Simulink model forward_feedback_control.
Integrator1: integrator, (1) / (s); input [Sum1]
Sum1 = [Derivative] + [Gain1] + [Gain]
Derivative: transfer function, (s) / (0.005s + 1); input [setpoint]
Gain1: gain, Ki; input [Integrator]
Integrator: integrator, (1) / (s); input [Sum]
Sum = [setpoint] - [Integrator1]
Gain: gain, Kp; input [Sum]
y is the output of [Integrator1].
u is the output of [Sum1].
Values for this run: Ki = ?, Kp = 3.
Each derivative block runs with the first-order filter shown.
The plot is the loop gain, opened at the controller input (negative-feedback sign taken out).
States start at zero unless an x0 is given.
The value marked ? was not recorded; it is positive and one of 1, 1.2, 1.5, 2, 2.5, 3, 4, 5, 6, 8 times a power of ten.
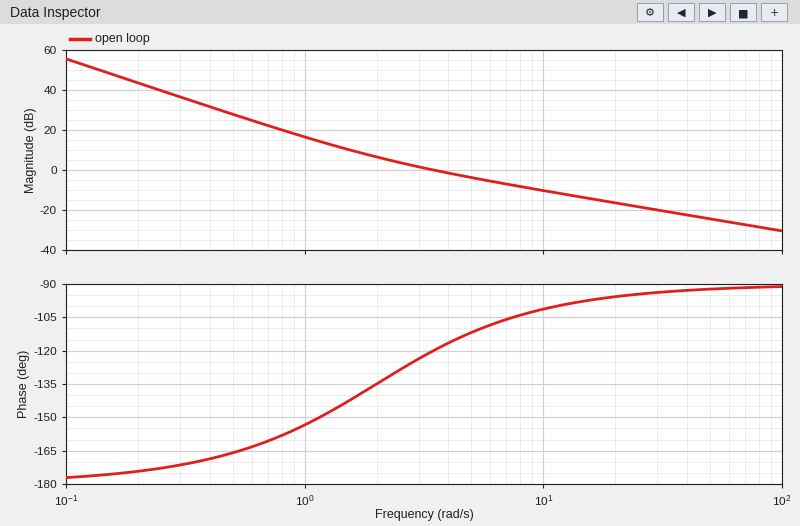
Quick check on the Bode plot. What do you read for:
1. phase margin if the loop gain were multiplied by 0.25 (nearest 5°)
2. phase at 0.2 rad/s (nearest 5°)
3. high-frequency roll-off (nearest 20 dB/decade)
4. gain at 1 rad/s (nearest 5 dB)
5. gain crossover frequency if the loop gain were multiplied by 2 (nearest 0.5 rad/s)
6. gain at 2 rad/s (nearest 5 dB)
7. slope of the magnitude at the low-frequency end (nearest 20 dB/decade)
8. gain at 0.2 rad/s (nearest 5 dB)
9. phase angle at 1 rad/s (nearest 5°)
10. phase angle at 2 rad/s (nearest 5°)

35°
-175°
-20 dB/decade
15 dB
6.5 rad/s
5 dB
-40 dB/decade
45 dB
-155°
-135°
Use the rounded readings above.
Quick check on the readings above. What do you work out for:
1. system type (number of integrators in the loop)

2
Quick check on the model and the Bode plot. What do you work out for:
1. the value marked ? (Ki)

6
